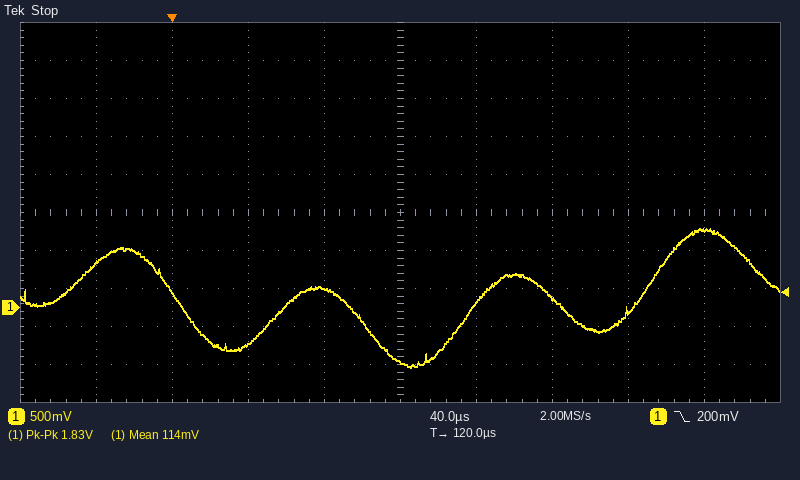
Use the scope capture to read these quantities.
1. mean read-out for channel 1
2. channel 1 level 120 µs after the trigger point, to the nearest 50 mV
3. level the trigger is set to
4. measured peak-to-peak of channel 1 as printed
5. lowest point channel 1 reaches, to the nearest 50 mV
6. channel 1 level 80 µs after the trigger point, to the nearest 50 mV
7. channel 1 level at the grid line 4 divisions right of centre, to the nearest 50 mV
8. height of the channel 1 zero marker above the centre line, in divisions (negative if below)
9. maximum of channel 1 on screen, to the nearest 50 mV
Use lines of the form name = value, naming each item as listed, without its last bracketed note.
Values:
mean read-out for channel 1 = 114 mV
channel 1 level 120 µs after the trigger point, to the nearest 50 mV = -700 mV
level the trigger is set to = 200 mV
measured peak-to-peak of channel 1 as printed = 1.83 V
lowest point channel 1 reaches, to the nearest 50 mV = -800 mV
channel 1 level 80 µs after the trigger point, to the nearest 50 mV = 250 mV
channel 1 level at the grid line 4 divisions right of centre, to the nearest 50 mV = 1.00 V
height of the channel 1 zero marker above the centre line, in divisions = -2.5 div
maximum of channel 1 on screen, to the nearest 50 mV = 1.05 V
